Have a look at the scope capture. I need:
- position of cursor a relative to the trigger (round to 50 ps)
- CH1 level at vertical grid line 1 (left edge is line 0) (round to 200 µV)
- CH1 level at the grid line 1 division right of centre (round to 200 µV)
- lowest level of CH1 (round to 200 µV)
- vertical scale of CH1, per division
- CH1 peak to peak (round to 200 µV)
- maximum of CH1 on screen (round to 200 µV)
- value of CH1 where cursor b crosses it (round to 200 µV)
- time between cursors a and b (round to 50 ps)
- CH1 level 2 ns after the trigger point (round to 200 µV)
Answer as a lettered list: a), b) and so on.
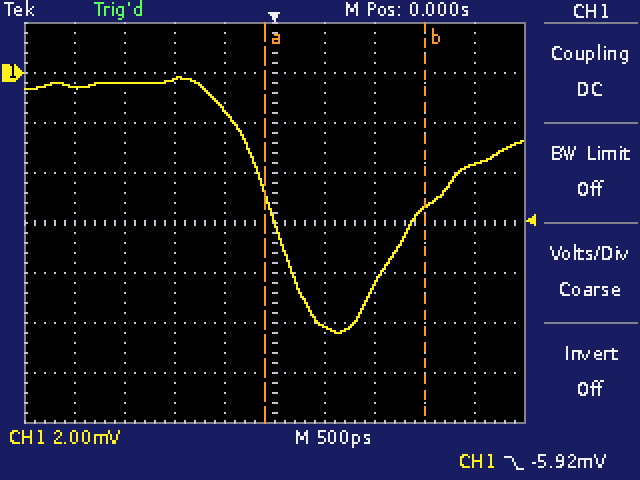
a) -100 ps
b) -600 µV
c) -10.2 mV
d) -10.4 mV
e) 2 mV
f) 10.2 mV
g) -200 µV
h) -5.4 mV
i) 1.60 ns
j) -3.6 mV
